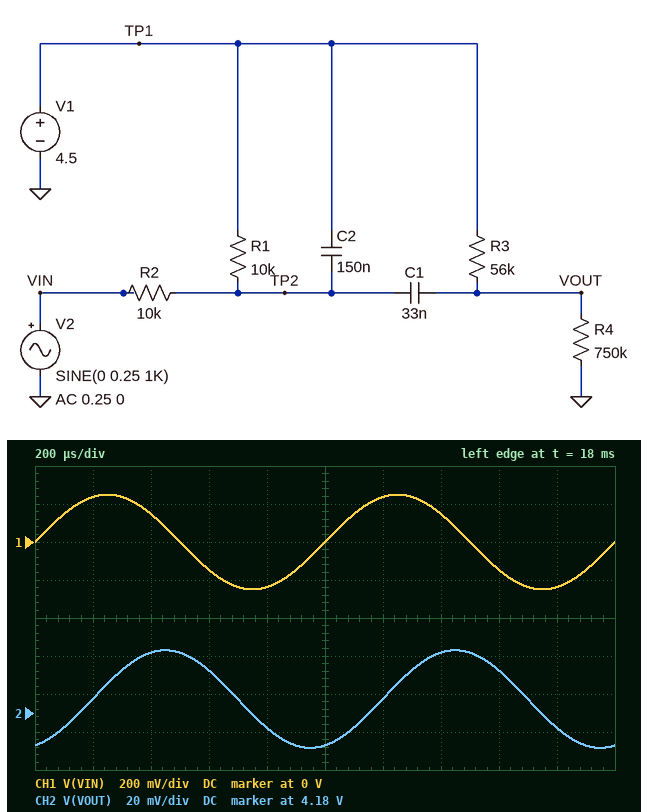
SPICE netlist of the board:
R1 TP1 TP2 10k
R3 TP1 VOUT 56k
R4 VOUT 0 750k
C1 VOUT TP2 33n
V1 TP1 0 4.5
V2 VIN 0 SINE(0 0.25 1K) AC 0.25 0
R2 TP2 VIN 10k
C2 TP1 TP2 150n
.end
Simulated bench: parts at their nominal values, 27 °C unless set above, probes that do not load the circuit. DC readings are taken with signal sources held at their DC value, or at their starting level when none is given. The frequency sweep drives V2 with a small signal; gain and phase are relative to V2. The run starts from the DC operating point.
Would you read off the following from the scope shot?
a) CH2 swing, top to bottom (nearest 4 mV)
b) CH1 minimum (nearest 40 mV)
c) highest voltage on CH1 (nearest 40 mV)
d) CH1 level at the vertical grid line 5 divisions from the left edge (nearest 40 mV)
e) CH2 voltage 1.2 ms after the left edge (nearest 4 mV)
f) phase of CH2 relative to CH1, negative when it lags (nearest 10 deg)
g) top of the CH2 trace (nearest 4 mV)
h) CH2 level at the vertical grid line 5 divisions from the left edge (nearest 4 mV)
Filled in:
52 mV
-240 mV
240 mV
0 V
4.188 V
-70 deg
4.212 V
4.164 V
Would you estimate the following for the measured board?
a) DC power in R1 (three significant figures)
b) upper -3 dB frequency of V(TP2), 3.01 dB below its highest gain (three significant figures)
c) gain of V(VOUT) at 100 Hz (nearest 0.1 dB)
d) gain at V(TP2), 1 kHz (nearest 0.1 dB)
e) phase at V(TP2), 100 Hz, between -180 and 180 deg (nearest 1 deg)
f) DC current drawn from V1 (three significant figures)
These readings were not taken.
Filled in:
506 µW
186 Hz
-10.1 dB
-19.7 dB
-26 deg
231 µA
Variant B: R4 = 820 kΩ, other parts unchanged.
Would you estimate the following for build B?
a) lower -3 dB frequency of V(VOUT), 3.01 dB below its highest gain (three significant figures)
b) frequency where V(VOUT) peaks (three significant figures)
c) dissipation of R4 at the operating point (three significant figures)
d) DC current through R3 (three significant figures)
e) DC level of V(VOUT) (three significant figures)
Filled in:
51.9 Hz
140 Hz
21.6 µW
5.14 µA
4.21 V
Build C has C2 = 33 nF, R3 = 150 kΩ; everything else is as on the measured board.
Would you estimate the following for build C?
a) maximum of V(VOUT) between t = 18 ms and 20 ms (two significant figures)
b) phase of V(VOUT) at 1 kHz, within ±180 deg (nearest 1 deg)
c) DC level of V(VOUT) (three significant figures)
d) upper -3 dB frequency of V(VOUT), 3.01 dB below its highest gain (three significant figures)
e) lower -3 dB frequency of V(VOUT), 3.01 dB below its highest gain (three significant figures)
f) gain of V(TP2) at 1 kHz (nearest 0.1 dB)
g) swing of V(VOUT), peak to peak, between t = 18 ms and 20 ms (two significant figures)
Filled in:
3.8 V
-43 deg
3.75 V
1.08 kHz
34.6 Hz
-9.4 dB
170 mV
